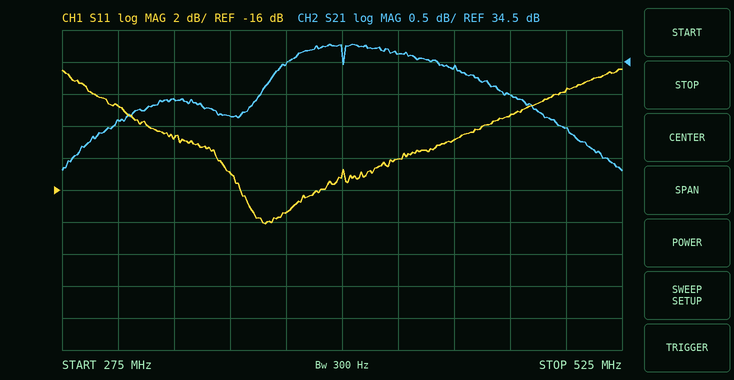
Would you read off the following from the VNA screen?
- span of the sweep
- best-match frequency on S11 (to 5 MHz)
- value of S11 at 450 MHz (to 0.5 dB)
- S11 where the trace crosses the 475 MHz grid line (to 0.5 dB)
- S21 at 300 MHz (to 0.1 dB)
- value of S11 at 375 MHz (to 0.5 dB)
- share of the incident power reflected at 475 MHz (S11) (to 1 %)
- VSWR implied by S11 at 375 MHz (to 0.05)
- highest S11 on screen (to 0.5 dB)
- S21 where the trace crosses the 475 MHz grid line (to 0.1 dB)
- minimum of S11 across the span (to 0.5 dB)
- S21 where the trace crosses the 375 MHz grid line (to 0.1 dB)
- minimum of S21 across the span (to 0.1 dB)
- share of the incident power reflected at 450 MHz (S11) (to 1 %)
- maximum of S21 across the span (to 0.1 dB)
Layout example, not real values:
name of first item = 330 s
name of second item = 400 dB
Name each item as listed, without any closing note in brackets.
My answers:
span of the sweep = 250 MHz
best-match frequency on S11 = 365 MHz
value of S11 at 450 MHz = -13.0 dB
S11 where the trace crosses the 475 MHz grid line = -11.5 dB
S21 at 300 MHz = 33.6 dB
value of S11 at 375 MHz = -17.5 dB
share of the incident power reflected at 475 MHz (S11) = 7 %
VSWR implied by S11 at 375 MHz = 1.30
highest S11 on screen = -8.5 dB
S21 where the trace crosses the 475 MHz grid line = 34.0 dB
minimum of S11 across the span = -18.0 dB
S21 where the trace crosses the 375 MHz grid line = 34.5 dB
minimum of S21 across the span = 32.8 dB
share of the incident power reflected at 450 MHz (S11) = 5 %
maximum of S21 across the span = 34.8 dB
